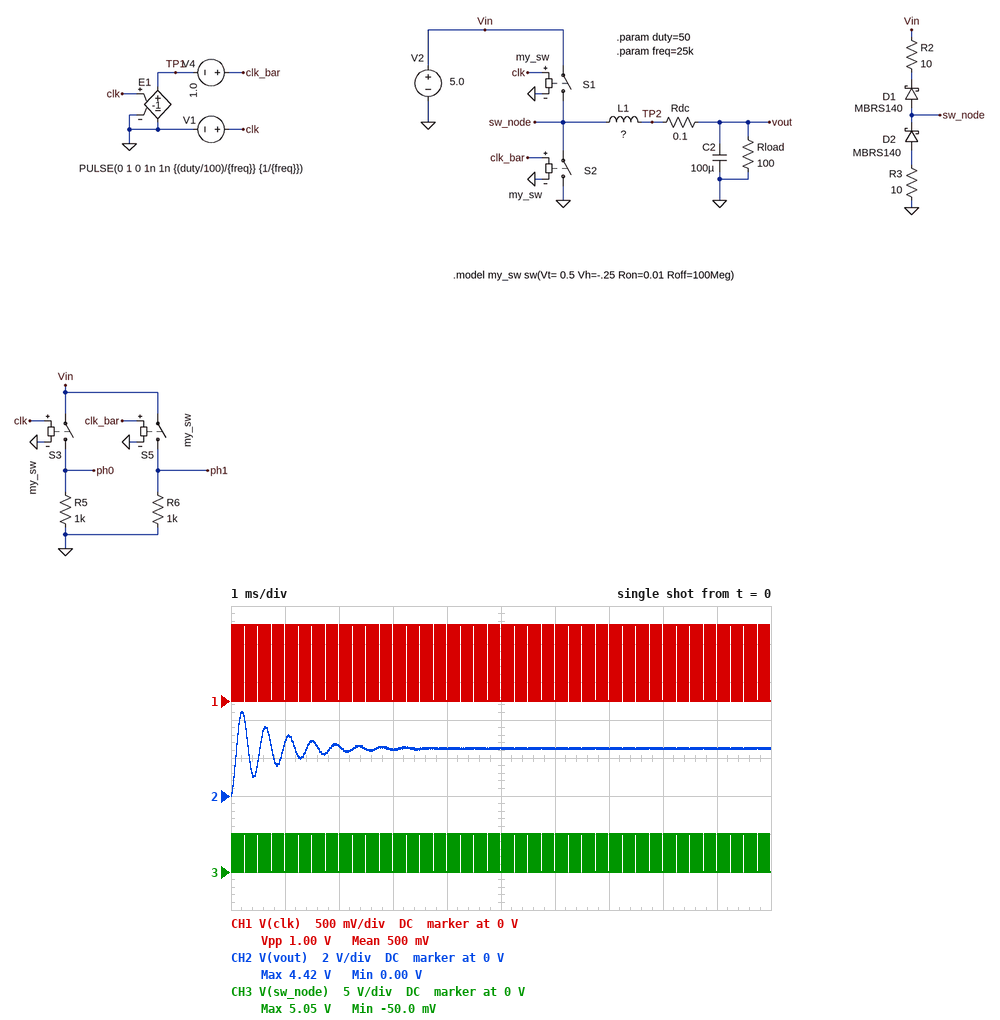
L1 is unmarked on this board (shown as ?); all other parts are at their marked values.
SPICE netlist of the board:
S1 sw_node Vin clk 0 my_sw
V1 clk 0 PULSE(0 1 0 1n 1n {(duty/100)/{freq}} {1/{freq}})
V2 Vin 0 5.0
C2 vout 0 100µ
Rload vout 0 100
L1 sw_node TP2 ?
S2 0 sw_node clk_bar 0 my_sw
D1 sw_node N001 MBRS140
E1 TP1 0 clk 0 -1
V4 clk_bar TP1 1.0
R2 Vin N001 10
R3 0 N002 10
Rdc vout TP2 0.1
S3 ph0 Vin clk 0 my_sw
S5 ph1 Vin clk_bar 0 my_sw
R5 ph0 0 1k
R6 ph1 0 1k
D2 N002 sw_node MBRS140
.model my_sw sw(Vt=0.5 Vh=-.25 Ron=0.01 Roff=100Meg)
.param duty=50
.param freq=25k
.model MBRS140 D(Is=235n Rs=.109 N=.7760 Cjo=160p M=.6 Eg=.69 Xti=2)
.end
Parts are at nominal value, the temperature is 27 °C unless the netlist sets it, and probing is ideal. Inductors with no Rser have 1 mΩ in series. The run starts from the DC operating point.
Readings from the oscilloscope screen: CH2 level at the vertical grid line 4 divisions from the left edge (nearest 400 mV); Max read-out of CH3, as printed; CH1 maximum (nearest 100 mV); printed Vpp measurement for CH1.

2.4 V
5.05 V
1.0 V
1.00 V
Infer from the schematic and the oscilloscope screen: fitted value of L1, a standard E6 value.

47 µH
